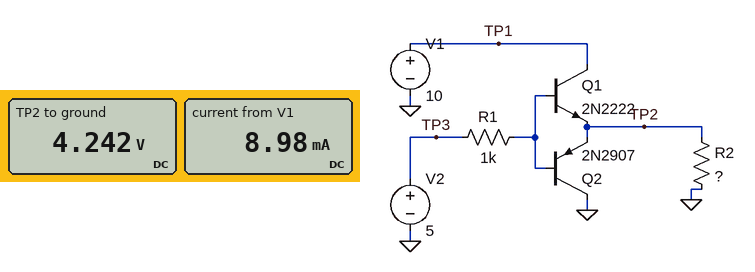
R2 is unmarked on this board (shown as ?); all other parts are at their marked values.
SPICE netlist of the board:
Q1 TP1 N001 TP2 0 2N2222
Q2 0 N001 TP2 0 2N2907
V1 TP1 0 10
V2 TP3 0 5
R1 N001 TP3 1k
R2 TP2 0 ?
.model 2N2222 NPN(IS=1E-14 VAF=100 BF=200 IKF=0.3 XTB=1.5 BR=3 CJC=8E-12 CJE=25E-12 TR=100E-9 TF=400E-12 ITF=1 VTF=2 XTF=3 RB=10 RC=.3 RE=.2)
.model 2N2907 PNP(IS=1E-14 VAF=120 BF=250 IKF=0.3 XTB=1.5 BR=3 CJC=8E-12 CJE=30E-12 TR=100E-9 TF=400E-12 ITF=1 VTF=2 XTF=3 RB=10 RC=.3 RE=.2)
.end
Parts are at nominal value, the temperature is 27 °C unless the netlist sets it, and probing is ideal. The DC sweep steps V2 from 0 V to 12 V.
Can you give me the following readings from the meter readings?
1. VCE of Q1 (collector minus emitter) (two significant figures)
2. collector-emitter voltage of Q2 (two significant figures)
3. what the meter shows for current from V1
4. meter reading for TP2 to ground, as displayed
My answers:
5.8 V
-4.2 V
8.98 mA
4.242 V
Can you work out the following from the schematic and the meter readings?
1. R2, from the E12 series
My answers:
470 Ω
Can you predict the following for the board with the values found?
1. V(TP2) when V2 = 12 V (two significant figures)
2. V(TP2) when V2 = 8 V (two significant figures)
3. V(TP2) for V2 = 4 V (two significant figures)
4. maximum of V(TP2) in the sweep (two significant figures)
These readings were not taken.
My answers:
9.9 V
7.2 V
3.3 V
9.9 V
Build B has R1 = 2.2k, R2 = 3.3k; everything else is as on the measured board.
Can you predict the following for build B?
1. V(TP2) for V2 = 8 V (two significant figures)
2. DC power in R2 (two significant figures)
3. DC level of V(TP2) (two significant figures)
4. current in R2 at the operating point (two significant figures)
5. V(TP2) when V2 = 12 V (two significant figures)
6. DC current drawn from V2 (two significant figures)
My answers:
7.3 V
5.7 mW
4.3 V
1.3 mA
10 V
6.2 µA
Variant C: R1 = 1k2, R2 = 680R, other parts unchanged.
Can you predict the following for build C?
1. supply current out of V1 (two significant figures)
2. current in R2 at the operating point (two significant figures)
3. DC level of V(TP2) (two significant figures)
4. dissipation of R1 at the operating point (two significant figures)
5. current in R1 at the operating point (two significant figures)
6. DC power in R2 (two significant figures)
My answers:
6.2 mA
6.3 mA
4.3 V
1.1 µW
30 µA
27 mW
